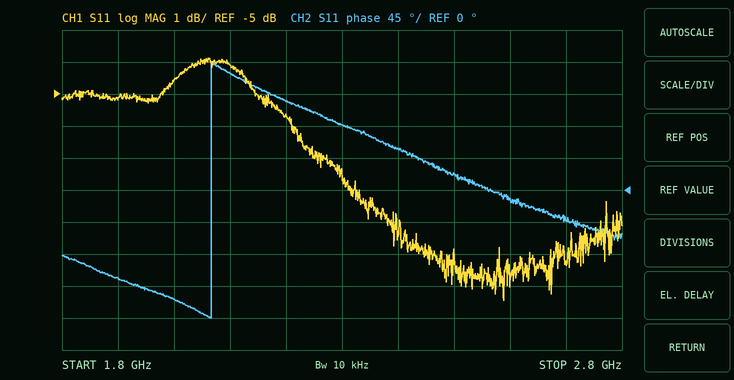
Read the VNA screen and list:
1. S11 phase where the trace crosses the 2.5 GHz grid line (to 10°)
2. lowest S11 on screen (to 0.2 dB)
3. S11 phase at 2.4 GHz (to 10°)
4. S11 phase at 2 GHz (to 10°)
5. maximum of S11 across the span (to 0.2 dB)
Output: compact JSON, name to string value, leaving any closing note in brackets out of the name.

{"S11 phase where the trace crosses the 2.5 GHz grid line": "20°", "lowest S11 on screen": "-11.4 dB", "S11 phase at 2.4 GHz": "60°", "S11 phase at 2 GHz": "-150°", "maximum of S11 across the span": "-3.8 dB"}
